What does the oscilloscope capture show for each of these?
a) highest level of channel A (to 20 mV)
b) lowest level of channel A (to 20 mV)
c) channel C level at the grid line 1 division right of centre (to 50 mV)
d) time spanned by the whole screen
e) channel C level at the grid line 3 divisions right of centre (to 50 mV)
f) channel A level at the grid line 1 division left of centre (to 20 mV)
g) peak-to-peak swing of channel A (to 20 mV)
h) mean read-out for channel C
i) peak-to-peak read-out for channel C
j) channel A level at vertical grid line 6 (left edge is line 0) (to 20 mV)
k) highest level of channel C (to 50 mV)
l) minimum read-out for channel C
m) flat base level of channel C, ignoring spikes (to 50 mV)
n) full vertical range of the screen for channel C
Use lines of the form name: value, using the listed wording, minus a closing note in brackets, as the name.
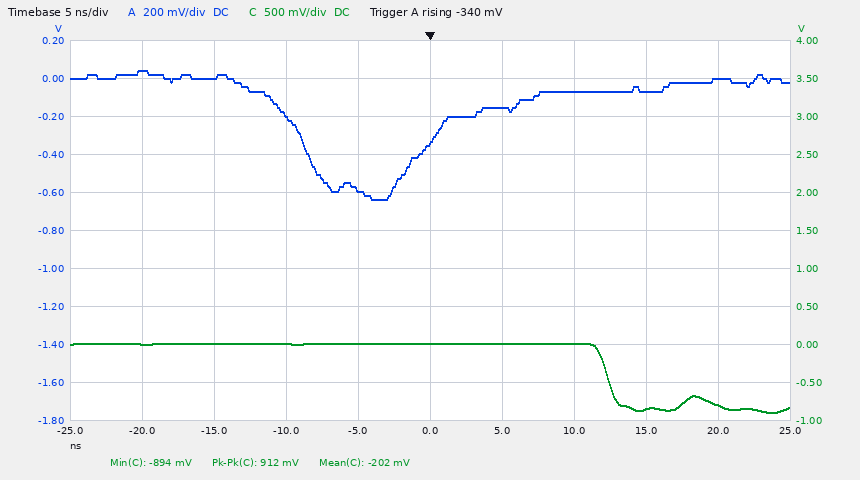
highest level of channel A: 40 mV
lowest level of channel A: -640 mV
channel C level at the grid line 1 division right of centre: 0 mV
time spanned by the whole screen: 50 ns
channel C level at the grid line 3 divisions right of centre: -850 mV
channel A level at the grid line 1 division left of centre: -580 mV
peak-to-peak swing of channel A: 680 mV
mean read-out for channel C: -202 mV
peak-to-peak read-out for channel C: 912 mV
channel A level at vertical grid line 6 (left edge is line 0): -160 mV
highest level of channel C: 0 mV
minimum read-out for channel C: -894 mV
flat base level of channel C, ignoring spikes: -850 mV
full vertical range of the screen for channel C: 5 V
